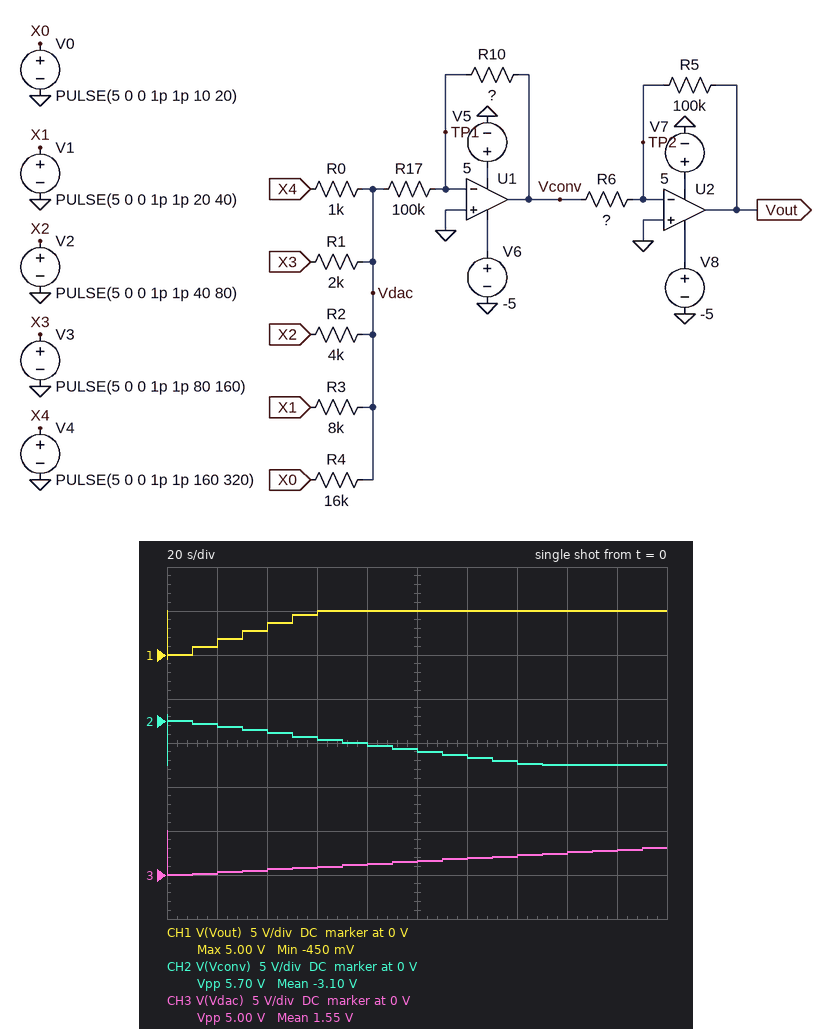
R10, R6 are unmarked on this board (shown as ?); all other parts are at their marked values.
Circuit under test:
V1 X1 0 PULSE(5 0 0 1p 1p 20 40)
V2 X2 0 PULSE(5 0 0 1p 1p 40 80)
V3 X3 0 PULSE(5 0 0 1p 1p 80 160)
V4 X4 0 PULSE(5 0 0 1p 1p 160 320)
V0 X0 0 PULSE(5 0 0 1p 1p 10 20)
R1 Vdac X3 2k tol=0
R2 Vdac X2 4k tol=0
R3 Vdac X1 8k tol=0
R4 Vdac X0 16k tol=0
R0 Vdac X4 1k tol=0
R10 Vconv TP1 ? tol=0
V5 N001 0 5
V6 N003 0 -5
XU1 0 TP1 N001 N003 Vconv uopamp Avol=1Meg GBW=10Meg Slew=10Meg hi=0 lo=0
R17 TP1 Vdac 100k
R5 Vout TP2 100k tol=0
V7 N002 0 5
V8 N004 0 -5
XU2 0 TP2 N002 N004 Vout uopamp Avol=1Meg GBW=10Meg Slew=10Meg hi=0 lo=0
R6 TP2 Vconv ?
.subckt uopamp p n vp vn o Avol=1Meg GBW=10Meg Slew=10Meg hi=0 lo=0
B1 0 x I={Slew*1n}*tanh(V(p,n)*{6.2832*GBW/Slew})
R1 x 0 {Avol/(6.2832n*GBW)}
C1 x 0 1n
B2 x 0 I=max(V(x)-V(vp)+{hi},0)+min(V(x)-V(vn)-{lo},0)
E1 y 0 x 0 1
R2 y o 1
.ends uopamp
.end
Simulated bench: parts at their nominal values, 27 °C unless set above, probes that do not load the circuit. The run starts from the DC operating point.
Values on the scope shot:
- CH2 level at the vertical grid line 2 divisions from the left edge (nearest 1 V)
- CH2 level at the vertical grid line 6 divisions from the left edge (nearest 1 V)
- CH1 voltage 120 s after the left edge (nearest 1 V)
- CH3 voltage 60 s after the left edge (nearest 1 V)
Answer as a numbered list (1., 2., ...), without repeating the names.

1. -1 V
2. -4 V
3. 5 V
4. 1 V
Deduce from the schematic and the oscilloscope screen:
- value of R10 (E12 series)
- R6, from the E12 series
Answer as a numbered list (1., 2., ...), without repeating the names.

1. 220 kΩ
2. 39 kΩ
